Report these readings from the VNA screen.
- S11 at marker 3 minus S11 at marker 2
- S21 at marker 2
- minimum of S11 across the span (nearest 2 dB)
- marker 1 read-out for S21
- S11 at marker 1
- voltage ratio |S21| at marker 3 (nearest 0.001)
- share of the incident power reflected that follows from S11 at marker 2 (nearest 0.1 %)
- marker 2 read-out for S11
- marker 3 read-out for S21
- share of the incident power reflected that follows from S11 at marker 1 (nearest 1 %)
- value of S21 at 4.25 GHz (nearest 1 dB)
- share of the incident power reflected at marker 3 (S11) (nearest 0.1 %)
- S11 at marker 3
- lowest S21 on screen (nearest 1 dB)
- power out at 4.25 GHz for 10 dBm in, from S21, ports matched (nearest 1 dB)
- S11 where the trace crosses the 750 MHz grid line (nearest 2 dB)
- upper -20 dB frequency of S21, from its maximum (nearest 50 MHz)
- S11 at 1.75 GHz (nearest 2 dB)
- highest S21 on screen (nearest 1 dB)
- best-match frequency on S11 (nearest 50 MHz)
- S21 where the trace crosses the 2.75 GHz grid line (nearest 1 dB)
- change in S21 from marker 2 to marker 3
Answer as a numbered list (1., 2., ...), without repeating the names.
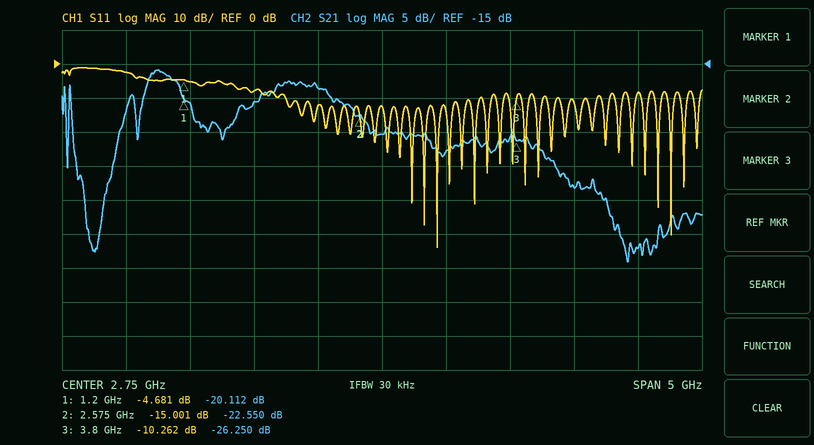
1. 4.739 dB
2. -22.550 dB
3. -54 dB
4. -20.112 dB
5. -4.681 dB
6. 0.049
7. 3.2 %
8. -15.001 dB
9. -26.250 dB
10. 34 %
11. -33 dB
12. 9.4 %
13. -10.262 dB
14. -44 dB
15. -23 dBm
16. -2 dB
17. 4.50 GHz
18. -8 dB
19. -16 dB
20. 3.20 GHz
21. -25 dB
22. -3.700 dB
